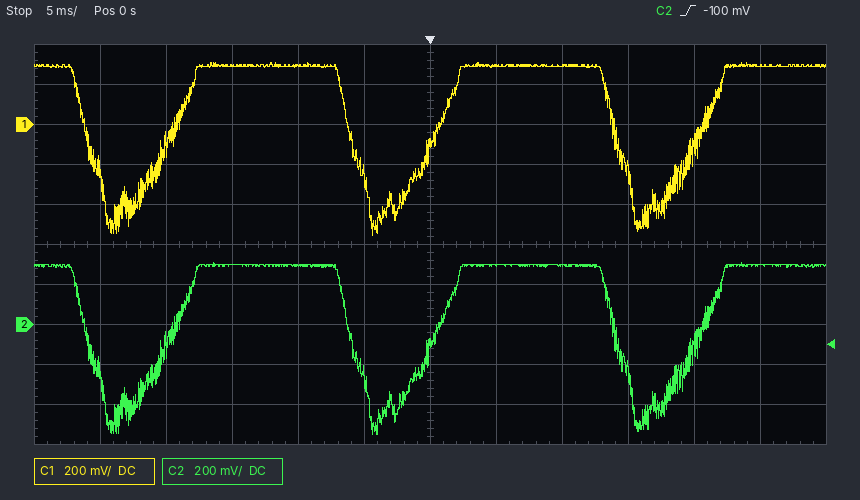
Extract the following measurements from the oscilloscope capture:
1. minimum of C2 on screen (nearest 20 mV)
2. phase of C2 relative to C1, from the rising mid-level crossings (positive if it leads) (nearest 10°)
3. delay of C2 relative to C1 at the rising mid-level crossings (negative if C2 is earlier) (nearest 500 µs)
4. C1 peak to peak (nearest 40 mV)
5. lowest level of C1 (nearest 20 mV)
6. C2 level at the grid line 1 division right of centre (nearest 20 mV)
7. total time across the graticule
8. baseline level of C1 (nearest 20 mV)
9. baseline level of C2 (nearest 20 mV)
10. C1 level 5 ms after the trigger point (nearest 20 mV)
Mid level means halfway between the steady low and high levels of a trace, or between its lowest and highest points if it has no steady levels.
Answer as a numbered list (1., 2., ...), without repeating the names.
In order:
1. -560 mV
2. 0°
3. 0.0 ms
4. 880 mV
5. -560 mV
6. 300 mV
7. 60 ms
8. 300 mV
9. 300 mV
10. 300 mV
